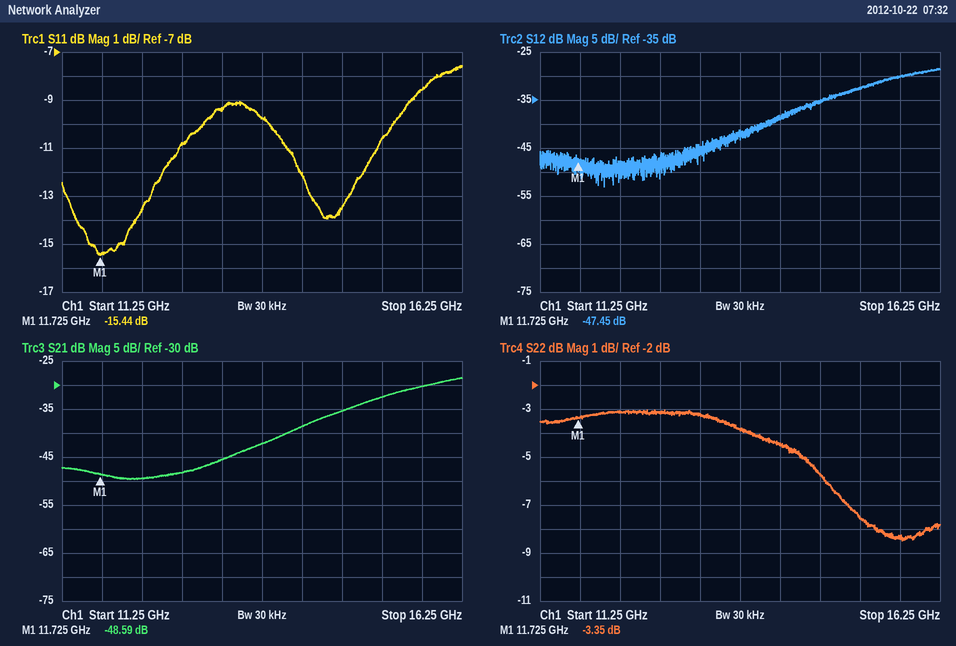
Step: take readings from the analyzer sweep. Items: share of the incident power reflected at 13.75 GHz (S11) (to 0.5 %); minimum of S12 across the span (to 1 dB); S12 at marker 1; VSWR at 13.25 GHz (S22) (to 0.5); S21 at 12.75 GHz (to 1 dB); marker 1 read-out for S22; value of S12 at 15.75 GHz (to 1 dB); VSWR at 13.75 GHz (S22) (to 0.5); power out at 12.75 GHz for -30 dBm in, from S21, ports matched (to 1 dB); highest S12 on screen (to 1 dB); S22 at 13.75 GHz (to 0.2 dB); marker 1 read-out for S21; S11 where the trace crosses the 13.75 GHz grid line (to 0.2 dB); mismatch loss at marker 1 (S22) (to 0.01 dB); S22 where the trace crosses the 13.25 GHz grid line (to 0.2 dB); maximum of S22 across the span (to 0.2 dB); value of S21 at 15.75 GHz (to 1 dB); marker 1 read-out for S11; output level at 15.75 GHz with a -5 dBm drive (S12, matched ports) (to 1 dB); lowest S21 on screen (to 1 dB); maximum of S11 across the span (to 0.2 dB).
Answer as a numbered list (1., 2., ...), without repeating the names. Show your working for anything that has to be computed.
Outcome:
1. 10^(-9.8/10) ≈ 10.5 %
2. -53 dB
3. -47.45 dB
4. |Γ| = 10^(-3.2/20) = 0.6918; VSWR = (1 + 0.6918)/(1 − 0.6918) ≈ 5.5
5. -48 dB
6. -3.35 dB
7. -30 dB
8. |Γ| = 10^(-3.8/20) = 0.6457; VSWR = (1 + 0.6457)/(1 − 0.6457) ≈ 4.64, so 4.5 to the nearest 0.5
9. -30 dBm + (-48 dB) = -78 dBm
10. -28 dB
11. -3.8 dB
12. -48.59 dB
13. -9.8 dB
14. −10 log10(1 − 10^(-3.35/10)) ≈ 2.70 dB
15. -3.2 dB
16. -3.0 dB
17. -30 dB
18. -15.44 dB
19. -5 dBm + (-30 dB) = -35 dBm
20. -50 dB
21. -7.6 dB
